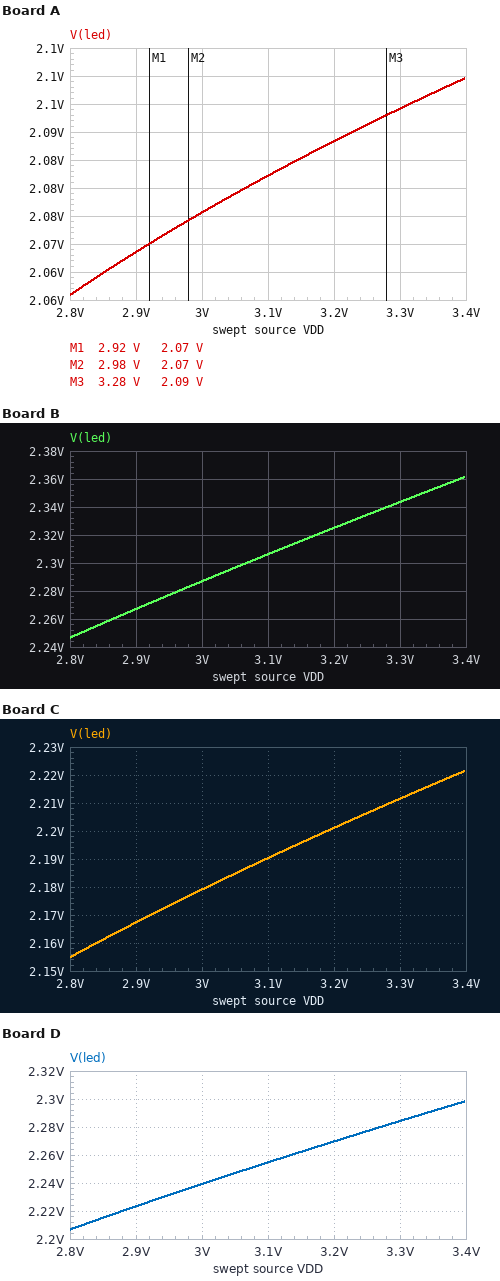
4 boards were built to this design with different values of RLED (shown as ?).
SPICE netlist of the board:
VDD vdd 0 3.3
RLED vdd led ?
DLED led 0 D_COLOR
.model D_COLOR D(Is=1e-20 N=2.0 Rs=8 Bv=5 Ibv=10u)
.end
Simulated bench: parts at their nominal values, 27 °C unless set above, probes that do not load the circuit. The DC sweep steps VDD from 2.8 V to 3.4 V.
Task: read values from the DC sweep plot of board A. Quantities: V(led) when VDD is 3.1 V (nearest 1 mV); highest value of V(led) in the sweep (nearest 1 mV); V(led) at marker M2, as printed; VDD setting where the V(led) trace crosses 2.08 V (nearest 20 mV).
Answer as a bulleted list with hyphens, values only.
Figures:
- 2.082 V
- 2.100 V
- 2.07 V
- 3.06 V
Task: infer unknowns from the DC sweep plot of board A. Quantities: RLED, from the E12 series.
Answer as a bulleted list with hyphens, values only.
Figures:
- 470 Ω
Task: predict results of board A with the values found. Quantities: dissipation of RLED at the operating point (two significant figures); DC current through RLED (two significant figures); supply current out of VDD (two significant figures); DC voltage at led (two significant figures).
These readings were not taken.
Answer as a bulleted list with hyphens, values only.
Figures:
- 3.1 mW
- 2.6 mA
- 2.6 mA
- 2.1 V
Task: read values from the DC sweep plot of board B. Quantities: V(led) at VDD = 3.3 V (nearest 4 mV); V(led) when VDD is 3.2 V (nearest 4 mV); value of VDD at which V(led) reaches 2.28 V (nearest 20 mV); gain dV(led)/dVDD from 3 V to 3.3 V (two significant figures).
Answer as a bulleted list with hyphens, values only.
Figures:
- 2.344 V
- 2.324 V
- 2.96 V
- 0.19 V/V
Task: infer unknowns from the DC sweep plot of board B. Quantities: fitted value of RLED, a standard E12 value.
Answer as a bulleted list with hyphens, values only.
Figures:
- 47 Ω
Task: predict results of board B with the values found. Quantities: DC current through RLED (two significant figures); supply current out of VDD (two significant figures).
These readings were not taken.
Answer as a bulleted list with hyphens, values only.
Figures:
- 20 mA
- 20 mA
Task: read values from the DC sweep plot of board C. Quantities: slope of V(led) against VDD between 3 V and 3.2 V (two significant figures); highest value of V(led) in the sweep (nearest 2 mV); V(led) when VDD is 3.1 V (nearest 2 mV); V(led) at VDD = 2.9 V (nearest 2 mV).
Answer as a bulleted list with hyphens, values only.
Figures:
- 0.11 V/V
- 2.222 V
- 2.190 V
- 2.168 V
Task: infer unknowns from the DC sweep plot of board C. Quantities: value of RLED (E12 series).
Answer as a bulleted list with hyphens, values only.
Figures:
- 120 Ω
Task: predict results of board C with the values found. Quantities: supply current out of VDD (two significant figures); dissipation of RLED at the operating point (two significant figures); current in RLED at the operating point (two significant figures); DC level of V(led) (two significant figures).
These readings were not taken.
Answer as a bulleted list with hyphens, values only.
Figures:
- 9.1 mA
- 9.9 mW
- 9.1 mA
- 2.2 V
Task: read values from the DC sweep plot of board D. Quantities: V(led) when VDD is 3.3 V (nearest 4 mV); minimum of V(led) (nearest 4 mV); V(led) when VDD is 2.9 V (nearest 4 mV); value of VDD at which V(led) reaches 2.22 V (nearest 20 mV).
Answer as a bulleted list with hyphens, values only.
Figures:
- 2.284 V
- 2.208 V
- 2.224 V
- 2.88 V
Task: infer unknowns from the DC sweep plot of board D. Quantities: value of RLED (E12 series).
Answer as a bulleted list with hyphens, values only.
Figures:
- 68 Ω
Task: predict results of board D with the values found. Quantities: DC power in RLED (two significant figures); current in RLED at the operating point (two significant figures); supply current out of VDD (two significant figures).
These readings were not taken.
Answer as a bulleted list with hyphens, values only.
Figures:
- 15 mW
- 15 mA
- 15 mA
